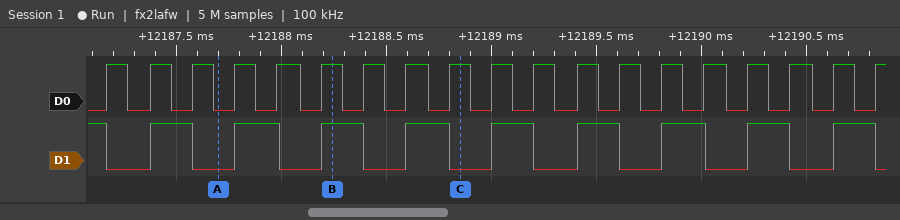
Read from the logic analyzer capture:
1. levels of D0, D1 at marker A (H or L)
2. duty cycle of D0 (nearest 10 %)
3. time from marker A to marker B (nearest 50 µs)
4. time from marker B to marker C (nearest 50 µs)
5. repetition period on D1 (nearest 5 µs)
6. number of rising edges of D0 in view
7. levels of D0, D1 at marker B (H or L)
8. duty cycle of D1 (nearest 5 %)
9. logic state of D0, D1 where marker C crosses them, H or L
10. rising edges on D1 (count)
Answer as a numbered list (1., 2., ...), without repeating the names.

1. D0=L, D1=L
2. 50 %
3. 550 µs
4. 600 µs
5. 405 µs
6. 19
7. D0=H, D1=H
8. 50 %
9. D0=H, D1=L
10. 9
